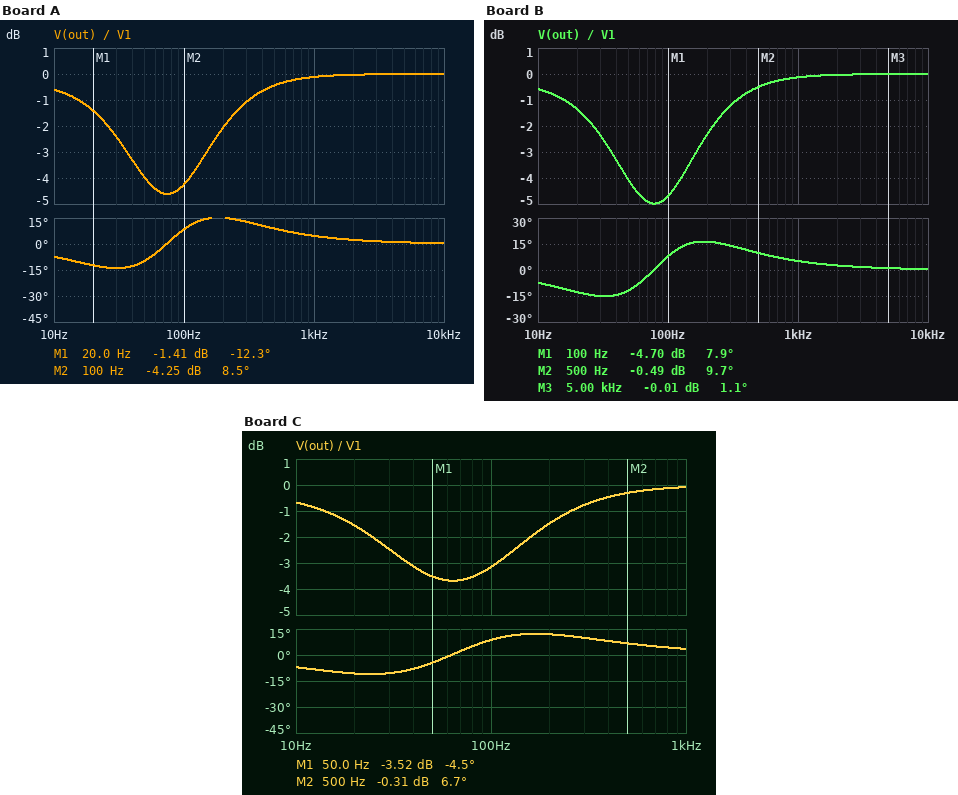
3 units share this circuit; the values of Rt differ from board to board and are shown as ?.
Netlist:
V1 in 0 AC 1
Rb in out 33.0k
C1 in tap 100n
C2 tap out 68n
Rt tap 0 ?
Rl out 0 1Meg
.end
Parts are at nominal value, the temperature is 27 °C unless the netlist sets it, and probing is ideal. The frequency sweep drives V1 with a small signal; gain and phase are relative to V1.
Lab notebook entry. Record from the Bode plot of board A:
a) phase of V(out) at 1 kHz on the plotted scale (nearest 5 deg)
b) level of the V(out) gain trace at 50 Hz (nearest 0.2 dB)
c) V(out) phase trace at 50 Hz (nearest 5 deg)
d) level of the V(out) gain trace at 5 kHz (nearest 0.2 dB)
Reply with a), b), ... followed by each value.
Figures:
a) 5 deg
b) -4.0 dB
c) -10 deg
d) 0 dB
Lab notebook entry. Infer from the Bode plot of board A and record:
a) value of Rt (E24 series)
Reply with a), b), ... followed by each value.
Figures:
a) 20 kΩ
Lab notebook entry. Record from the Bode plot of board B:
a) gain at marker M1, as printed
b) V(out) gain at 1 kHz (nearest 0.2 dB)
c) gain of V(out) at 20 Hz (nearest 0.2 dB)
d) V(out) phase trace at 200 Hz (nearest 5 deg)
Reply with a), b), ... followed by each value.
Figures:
a) -4.70 dB
b) -0.2 dB
c) -1.4 dB
d) 15 deg
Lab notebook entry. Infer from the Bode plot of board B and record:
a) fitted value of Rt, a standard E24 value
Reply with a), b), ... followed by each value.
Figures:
a) 18 kΩ
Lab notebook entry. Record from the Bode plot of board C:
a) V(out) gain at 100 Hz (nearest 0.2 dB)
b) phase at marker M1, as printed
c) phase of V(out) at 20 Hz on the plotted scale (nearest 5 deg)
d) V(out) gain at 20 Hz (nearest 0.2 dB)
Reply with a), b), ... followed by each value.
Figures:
a) -3.2 dB
b) -4.5 deg
c) -10 deg
d) -1.6 dB
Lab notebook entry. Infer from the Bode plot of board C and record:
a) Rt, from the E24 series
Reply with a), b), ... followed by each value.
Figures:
a) 27 kΩ
